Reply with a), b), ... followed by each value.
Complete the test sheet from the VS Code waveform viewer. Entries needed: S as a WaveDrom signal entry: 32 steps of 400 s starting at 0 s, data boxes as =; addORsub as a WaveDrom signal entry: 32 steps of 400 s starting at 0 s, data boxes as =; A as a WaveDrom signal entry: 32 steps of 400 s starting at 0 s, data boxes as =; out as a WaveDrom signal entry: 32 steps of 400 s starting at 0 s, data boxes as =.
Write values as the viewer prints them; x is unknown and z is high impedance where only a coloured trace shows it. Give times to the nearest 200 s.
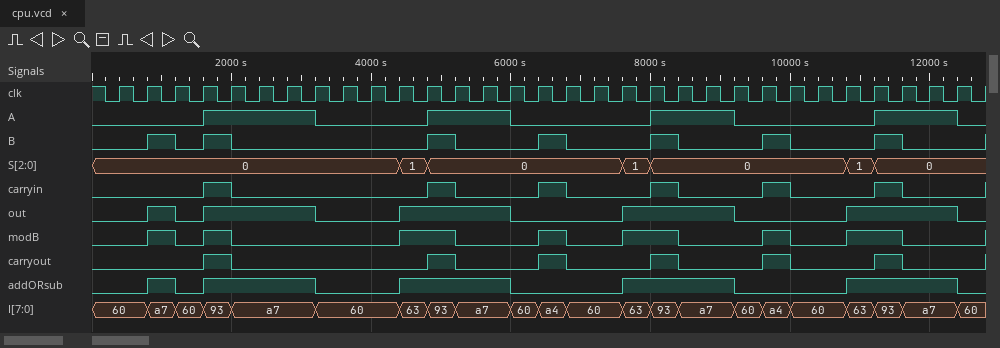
a) {name: 'S', wave: '=..........==......==......==...', data: '0 1 0 1 0 1 0'}
b) {name: 'addORsub', wave: '0.101...0..1...0...1...0...1...0'}
c) {name: 'A', wave: '0...1...0...1..0....1..0....1..0'}
d) {name: 'out', wave: '0.101...0..1...0...1...0...1...0'}
